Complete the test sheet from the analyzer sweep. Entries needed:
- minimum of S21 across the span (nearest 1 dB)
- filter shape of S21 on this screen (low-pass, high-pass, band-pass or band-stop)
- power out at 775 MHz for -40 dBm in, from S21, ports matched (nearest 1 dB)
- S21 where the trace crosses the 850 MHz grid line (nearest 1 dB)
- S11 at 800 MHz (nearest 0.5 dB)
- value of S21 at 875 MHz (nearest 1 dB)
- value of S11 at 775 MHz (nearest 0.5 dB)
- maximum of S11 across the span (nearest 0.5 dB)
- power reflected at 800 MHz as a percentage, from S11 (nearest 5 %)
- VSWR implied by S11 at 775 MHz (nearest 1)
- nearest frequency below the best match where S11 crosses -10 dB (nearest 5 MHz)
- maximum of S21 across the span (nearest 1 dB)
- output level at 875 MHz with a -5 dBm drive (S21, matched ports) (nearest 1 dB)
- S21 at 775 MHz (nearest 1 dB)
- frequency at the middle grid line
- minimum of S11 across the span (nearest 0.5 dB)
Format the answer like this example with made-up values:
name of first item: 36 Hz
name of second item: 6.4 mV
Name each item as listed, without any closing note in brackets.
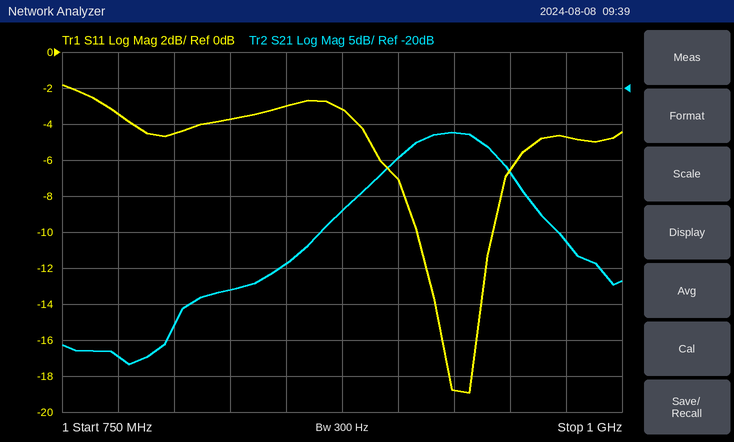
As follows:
minimum of S21 across the span: -58 dB
filter shape of S21 on this screen: band-pass
power out at 775 MHz for -40 dBm in, from S21, ports matched: -97 dBm
S21 where the trace crosses the 850 MHz grid line: -44 dB
S11 at 800 MHz: -4.5 dB
value of S21 at 875 MHz: -37 dB
value of S11 at 775 MHz: -3.5 dB
maximum of S11 across the span: -2.0 dB
power reflected at 800 MHz as a percentage, from S11: 35 %
VSWR implied by S11 at 775 MHz: 5
nearest frequency below the best match where S11 crosses -10 dB: 910 MHz
maximum of S21 across the span: -26 dB
output level at 875 MHz with a -5 dBm drive (S21, matched ports): -42 dBm
S21 at 775 MHz: -57 dB
frequency at the middle grid line: 875 MHz
minimum of S11 across the span: -19.0 dB
